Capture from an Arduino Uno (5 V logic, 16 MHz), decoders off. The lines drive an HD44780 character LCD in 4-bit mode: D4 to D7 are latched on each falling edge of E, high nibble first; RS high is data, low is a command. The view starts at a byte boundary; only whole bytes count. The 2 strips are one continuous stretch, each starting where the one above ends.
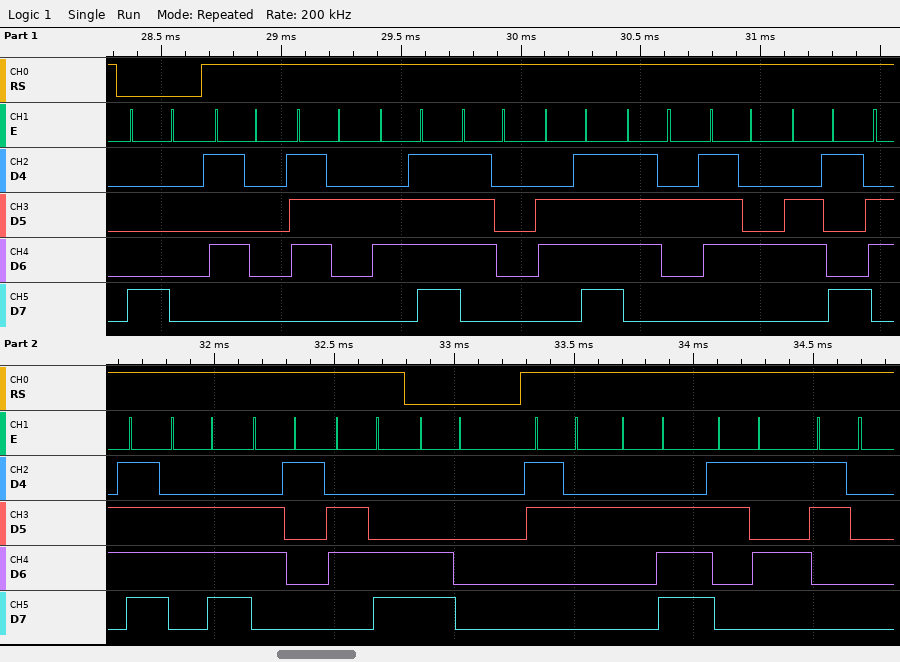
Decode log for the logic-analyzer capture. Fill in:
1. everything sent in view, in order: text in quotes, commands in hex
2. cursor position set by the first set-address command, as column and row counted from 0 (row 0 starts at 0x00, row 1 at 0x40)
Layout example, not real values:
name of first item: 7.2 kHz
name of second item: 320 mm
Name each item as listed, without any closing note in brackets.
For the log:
everything sent in view, in order: text in quotes, commands in hex: 0x80 "Proportional" 0xC0 "2.50"
cursor position set by the first set-address command, as column and row counted from 0: column 0, row 0
